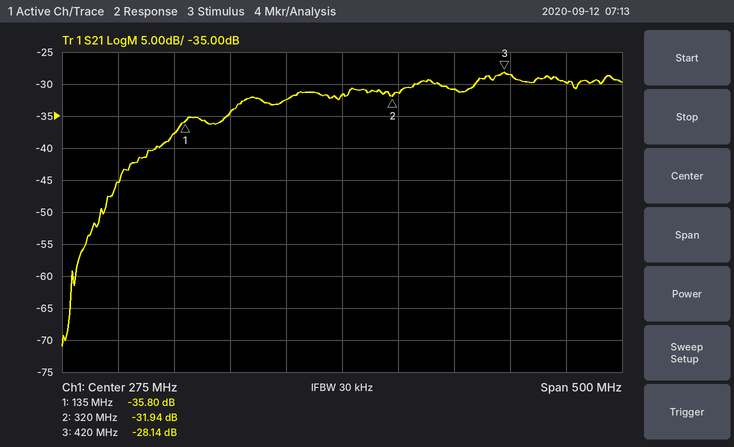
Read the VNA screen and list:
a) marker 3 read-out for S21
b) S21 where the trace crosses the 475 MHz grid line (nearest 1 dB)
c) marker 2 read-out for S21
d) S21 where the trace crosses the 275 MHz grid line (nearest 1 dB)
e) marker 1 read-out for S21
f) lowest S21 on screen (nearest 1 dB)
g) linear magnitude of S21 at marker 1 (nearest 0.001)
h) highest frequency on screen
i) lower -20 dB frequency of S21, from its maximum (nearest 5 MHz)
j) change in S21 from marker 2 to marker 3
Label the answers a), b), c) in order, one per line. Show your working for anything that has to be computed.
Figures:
a) -28.14 dB
b) -30 dB
c) -31.94 dB
d) -32 dB
e) -35.80 dB
f) -71 dB
g) 10^(-35.8/20) ≈ 0.016
h) 525 MHz
i) 65 MHz
j) -28.14 − (-31.94) = 3.80 dB
